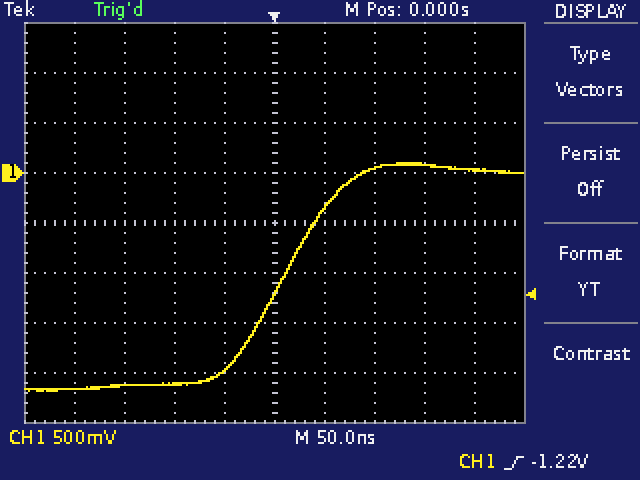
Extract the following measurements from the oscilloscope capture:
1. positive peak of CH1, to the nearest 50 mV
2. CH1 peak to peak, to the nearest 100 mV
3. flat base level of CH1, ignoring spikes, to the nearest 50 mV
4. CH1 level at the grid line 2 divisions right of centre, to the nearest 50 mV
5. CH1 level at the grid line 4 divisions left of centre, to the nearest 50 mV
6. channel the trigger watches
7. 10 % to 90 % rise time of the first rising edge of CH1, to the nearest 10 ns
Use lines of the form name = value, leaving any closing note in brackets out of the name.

positive peak of CH1, to the nearest 50 mV = 100 mV
CH1 peak to peak, to the nearest 100 mV = 2.30 V
flat base level of CH1, ignoring spikes, to the nearest 50 mV = -2.15 V
CH1 level at the grid line 2 divisions right of centre, to the nearest 50 mV = 50 mV
CH1 level at the grid line 4 divisions left of centre, to the nearest 50 mV = -2.15 V
channel the trigger watches = CH1
10 % to 90 % rise time of the first rising edge of CH1, to the nearest 10 ns = 110 ns
